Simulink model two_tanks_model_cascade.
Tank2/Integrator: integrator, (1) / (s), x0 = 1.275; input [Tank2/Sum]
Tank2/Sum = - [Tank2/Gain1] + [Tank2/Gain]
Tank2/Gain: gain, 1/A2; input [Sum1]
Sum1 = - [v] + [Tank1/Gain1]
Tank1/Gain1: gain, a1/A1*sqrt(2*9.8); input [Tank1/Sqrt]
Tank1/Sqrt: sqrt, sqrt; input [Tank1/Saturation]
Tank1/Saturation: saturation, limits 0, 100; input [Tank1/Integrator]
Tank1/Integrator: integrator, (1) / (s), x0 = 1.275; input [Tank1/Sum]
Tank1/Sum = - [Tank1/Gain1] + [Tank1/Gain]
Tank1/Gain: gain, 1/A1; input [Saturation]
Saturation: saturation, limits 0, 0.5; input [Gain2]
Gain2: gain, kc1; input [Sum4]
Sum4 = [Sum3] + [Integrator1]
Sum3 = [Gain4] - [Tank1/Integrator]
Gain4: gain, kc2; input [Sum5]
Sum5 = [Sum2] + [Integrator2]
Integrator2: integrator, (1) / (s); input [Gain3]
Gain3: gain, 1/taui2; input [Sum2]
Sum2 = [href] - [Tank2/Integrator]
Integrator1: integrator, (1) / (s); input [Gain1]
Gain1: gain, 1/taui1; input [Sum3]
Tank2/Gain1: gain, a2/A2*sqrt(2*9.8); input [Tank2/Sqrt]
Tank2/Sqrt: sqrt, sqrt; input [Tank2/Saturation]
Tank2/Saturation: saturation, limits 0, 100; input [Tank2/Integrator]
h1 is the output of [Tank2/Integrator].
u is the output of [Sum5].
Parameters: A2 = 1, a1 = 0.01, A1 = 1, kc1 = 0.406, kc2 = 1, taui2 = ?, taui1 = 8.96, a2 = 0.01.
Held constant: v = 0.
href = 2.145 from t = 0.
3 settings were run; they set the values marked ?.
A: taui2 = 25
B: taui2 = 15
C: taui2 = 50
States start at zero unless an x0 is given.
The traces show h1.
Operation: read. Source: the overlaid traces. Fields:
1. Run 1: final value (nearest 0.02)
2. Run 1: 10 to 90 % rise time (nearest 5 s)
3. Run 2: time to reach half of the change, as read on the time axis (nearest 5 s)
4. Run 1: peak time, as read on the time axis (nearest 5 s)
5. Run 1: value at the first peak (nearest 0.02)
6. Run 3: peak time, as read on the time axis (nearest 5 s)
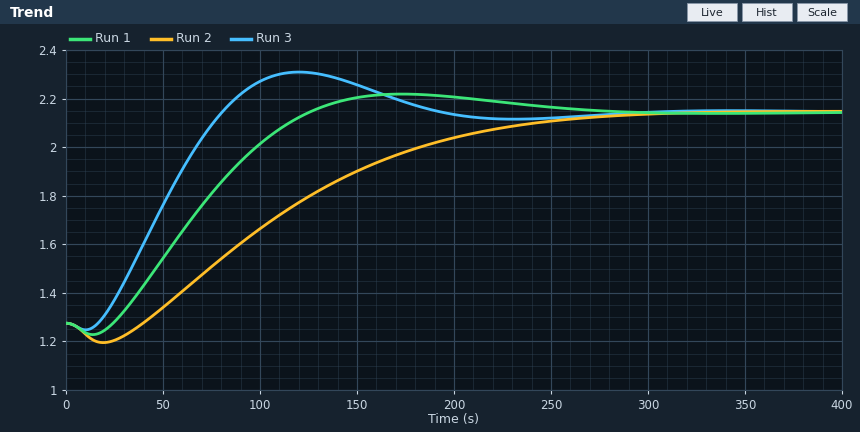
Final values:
2.14
75 s
110 s
175 s
2.22
120 s
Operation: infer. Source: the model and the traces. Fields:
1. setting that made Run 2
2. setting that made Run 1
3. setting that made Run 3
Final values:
C
A
B
